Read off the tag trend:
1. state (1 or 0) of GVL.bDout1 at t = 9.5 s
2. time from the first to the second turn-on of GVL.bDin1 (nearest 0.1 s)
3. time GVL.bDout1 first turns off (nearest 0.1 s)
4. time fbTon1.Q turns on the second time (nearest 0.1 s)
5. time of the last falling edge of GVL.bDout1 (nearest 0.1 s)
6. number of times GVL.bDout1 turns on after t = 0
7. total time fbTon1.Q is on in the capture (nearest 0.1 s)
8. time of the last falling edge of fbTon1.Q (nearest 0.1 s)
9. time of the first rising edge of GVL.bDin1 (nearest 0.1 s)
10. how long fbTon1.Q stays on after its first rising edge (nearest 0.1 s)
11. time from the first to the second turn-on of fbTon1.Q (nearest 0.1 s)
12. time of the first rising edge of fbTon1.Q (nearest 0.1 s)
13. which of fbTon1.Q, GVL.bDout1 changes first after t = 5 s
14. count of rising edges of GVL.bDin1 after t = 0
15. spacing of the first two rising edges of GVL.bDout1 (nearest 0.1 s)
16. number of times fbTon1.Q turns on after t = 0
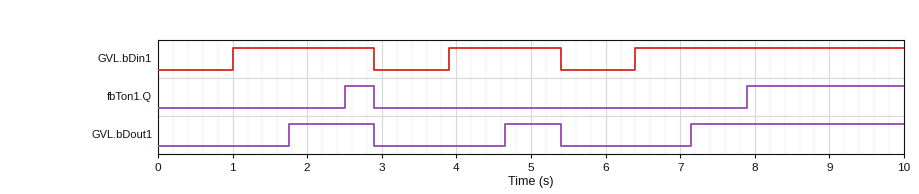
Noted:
1
2.9 s
2.9 s
7.9 s
5.4 s
3
2.5 s
2.9 s
1.0 s
0.4 s
5.4 s
2.5 s
GVL.bDout1
3
2.9 s
2
